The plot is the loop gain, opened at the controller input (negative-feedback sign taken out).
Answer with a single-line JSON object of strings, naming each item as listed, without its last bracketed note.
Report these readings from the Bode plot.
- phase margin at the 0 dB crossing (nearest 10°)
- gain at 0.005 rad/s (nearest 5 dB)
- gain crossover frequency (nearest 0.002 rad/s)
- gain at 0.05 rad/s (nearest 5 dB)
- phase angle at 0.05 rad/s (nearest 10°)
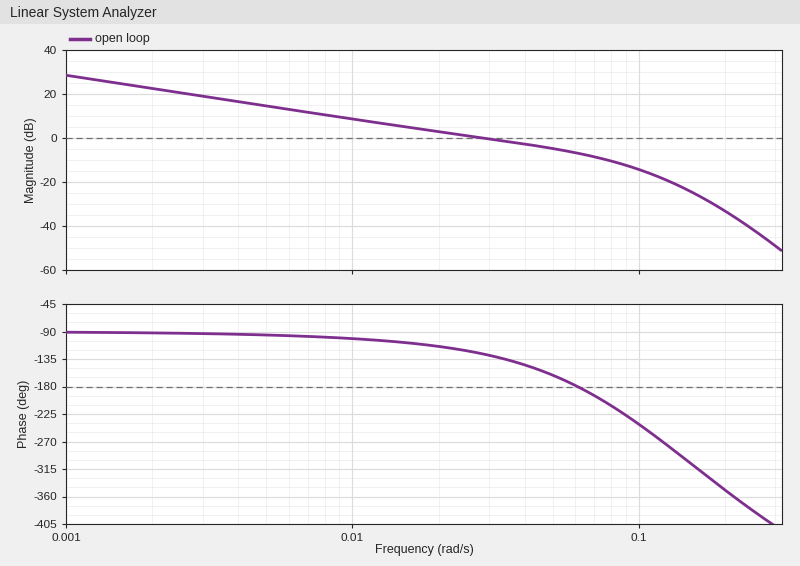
{"phase margin at the 0 dB crossing": "50°", "gain at 0.005 rad/s": "15 dB", "gain crossover frequency": "0.028 rad/s", "gain at 0.05 rad/s": "-5 dB", "phase angle at 0.05 rad/s": "-160°"}
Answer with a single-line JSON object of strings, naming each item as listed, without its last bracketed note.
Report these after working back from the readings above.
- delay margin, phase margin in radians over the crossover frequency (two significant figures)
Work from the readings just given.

{"delay margin, phase margin in radians over the crossover frequency": "31 s"}
